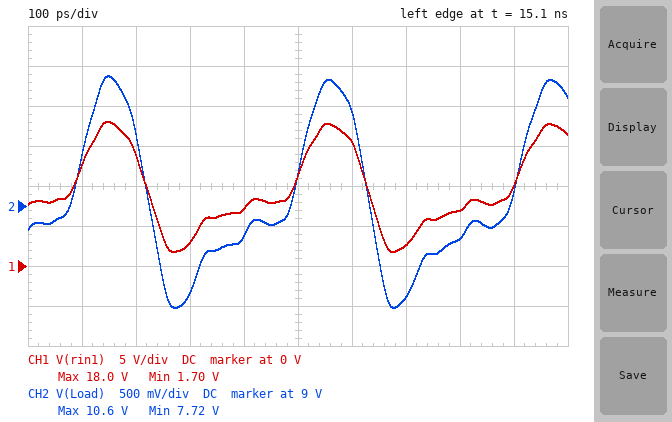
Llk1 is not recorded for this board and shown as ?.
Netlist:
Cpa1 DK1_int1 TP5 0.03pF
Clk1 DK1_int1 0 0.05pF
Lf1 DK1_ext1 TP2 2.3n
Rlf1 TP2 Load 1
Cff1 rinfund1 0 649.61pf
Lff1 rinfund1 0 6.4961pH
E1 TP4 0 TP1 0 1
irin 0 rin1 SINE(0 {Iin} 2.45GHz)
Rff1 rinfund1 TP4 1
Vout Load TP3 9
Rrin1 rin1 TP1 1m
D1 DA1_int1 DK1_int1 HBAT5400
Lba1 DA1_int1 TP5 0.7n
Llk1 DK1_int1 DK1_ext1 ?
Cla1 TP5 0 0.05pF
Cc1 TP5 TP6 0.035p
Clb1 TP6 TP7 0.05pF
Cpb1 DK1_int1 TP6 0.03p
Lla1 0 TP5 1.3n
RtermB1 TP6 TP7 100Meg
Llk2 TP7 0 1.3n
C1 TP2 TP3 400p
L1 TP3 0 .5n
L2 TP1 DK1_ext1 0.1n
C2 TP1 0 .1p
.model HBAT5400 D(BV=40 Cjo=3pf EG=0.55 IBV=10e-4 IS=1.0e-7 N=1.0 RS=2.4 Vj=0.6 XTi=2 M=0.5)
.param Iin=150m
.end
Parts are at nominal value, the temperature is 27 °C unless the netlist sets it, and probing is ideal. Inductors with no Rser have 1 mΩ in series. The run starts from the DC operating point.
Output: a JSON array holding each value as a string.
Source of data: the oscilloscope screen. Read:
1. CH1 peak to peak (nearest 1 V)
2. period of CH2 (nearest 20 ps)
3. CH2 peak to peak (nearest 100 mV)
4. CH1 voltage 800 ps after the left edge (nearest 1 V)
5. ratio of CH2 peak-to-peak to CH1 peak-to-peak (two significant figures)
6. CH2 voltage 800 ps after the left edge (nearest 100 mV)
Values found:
["16 V", "400 ps", "2.9 V", "7 V", "0.18", "8.6 V"]
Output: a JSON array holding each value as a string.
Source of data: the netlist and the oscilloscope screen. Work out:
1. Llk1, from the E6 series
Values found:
["470 pH"]
